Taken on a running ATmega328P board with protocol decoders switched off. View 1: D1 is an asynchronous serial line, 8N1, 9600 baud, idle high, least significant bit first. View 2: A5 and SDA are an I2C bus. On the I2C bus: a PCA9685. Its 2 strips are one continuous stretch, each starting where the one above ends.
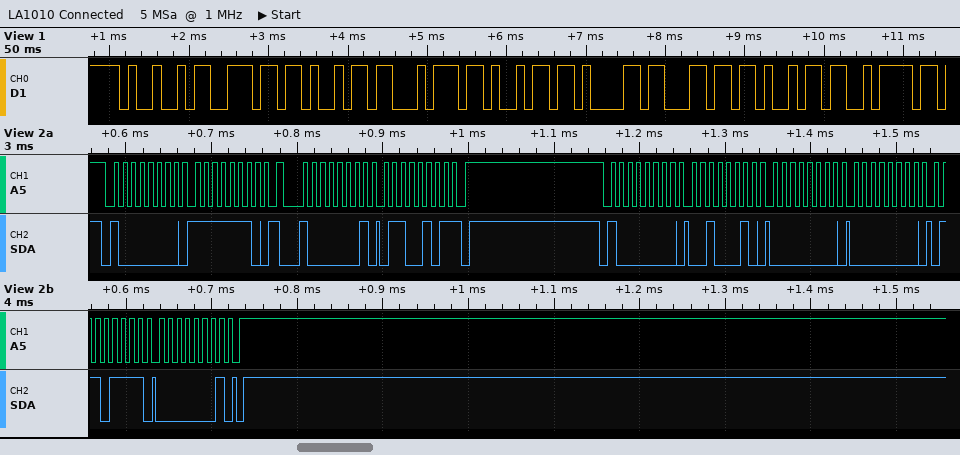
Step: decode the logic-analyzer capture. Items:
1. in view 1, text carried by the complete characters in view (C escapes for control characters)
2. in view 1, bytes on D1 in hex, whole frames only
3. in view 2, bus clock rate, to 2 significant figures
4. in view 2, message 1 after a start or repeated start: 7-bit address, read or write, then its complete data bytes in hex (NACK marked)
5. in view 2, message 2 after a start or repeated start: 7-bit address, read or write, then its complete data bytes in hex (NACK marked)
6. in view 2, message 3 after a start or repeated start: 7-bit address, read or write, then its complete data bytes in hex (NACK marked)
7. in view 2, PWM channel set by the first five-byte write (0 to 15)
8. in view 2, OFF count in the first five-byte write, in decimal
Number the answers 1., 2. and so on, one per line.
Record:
1. "Initializ"
2. 0x49 0x6E 0x69 0x74 0x69 0x61 0x6C 0x69 0x7A
3. 100 kHz
4. 0x40 write: FE
5. 0x40 read: 65 NACK
6. 0x40 write: 22 00 00 6F 01
7. 7
8. 367
